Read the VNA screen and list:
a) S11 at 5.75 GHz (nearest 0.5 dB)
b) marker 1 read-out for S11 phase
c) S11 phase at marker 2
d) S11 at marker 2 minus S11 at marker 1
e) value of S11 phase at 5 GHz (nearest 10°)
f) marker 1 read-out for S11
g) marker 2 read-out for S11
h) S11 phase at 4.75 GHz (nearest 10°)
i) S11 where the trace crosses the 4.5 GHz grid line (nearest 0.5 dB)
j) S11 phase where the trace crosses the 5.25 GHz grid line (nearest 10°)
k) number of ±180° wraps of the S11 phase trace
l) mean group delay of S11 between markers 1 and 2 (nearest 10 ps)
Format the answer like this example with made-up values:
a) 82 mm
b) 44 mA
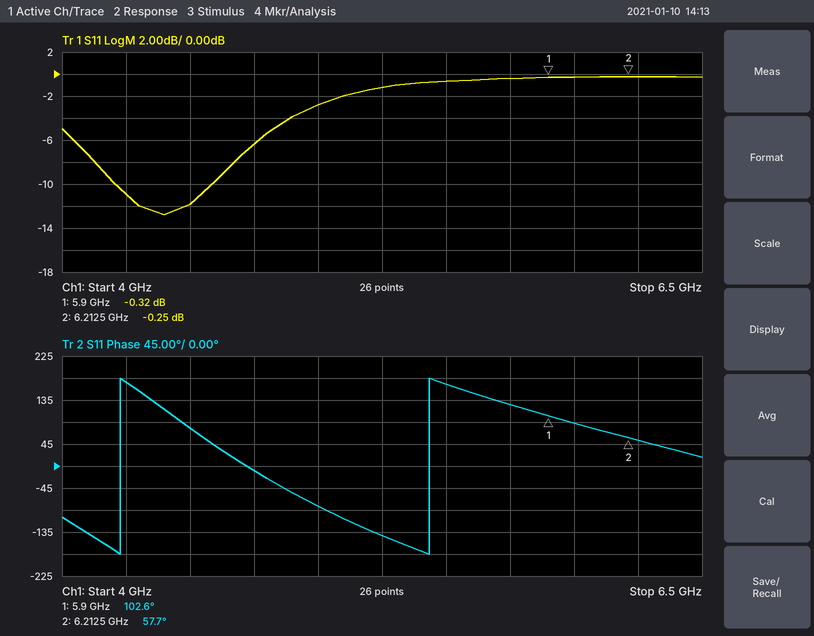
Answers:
a) -0.5 dB
b) 102.6°
c) 57.7°
d) 0.07 dB
e) -80°
f) -0.32 dB
g) -0.25 dB
h) -10°
i) -12.0 dB
j) -140°
k) 2
l) 400 ps
